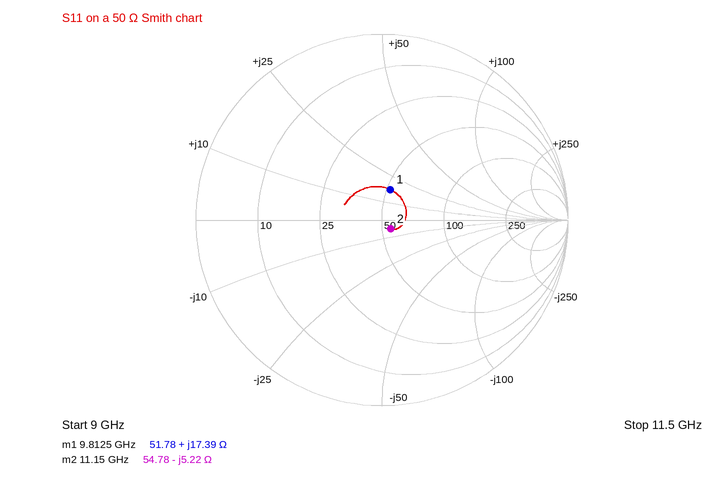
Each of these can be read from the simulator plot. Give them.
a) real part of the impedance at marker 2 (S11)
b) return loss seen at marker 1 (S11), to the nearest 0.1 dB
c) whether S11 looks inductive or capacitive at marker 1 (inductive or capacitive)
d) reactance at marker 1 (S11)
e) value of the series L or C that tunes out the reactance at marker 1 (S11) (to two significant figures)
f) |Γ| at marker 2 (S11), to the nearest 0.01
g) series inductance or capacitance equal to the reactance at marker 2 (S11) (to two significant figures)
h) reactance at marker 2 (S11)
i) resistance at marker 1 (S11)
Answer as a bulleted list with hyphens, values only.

- 54.78 Ω
- 15.4 dB
- inductive
- +17.39 Ω
- 930 fF
- 0.07
- 2.7 pF
- -5.22 Ω
- 51.78 Ω
